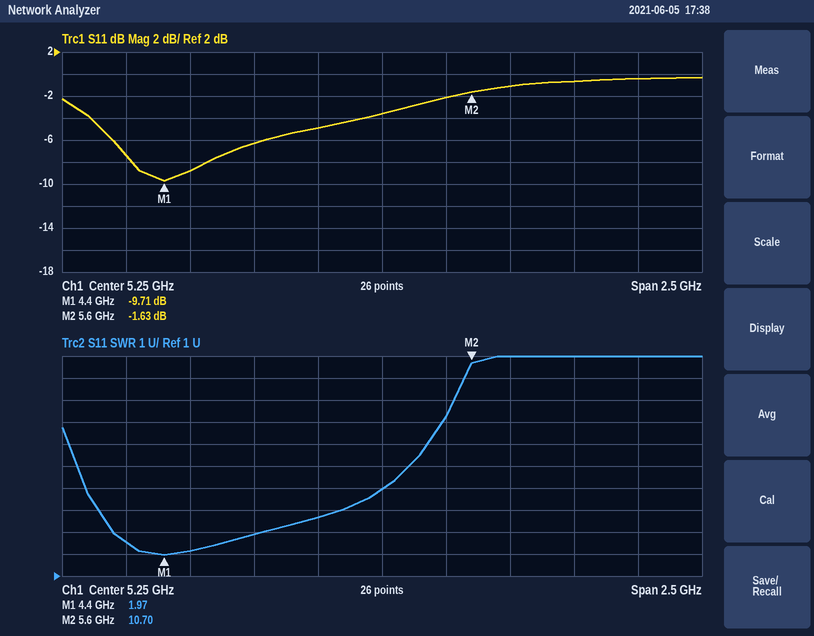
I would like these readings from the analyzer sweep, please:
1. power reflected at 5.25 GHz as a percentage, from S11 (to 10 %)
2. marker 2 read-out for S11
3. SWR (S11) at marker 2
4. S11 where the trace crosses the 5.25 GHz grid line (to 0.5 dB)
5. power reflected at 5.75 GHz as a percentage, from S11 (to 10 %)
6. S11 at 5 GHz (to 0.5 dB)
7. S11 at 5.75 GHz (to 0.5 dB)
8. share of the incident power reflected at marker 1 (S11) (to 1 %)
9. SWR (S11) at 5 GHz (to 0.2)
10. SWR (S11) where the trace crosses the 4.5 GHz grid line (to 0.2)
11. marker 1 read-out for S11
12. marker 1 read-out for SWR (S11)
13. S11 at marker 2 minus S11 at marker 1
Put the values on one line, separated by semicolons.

40 %; -1.63 dB; 10.70; -3.5 dB; 80 %; -5.0 dB; -1.0 dB; 11 %; 3.6; 2.2; -9.71 dB; 1.97; 8.08 dB
